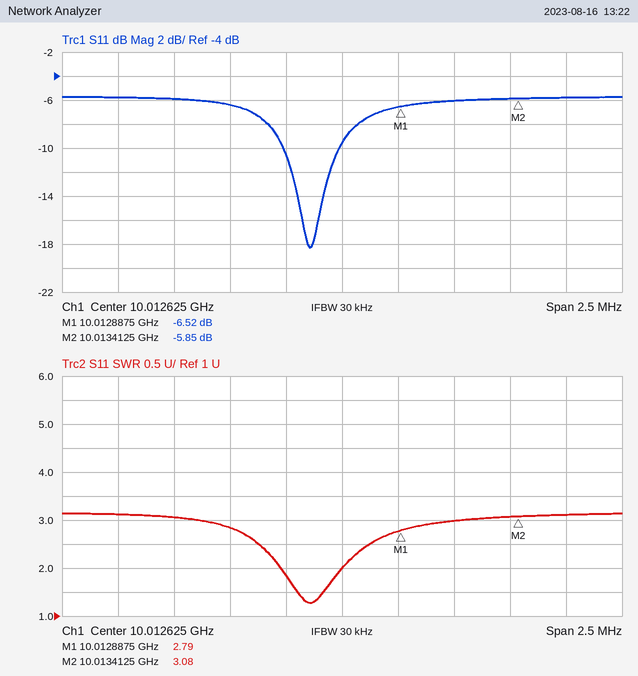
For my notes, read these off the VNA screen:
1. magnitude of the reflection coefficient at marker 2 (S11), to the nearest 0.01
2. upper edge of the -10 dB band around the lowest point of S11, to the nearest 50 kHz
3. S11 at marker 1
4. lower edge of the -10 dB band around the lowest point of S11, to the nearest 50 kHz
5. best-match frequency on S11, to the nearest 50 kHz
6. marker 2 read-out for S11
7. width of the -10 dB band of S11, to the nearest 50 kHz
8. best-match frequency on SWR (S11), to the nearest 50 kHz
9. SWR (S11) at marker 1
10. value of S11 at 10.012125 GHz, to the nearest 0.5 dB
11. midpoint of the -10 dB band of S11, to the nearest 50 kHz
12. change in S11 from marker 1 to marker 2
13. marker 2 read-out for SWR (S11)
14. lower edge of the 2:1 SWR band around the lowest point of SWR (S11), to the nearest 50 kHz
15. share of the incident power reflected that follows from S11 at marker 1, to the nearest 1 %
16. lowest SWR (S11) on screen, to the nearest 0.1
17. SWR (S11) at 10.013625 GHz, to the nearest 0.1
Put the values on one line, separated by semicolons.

0.51; 10.01260 GHz; -6.52 dB; 10.01235 GHz; 10.01250 GHz; -5.85 dB; 250 kHz; 10.01250 GHz; 2.79; -6.5 dB; 10.01250 GHz; 0.67 dB; 3.08; 10.01235 GHz; 22 %; 1.3; 3.1
